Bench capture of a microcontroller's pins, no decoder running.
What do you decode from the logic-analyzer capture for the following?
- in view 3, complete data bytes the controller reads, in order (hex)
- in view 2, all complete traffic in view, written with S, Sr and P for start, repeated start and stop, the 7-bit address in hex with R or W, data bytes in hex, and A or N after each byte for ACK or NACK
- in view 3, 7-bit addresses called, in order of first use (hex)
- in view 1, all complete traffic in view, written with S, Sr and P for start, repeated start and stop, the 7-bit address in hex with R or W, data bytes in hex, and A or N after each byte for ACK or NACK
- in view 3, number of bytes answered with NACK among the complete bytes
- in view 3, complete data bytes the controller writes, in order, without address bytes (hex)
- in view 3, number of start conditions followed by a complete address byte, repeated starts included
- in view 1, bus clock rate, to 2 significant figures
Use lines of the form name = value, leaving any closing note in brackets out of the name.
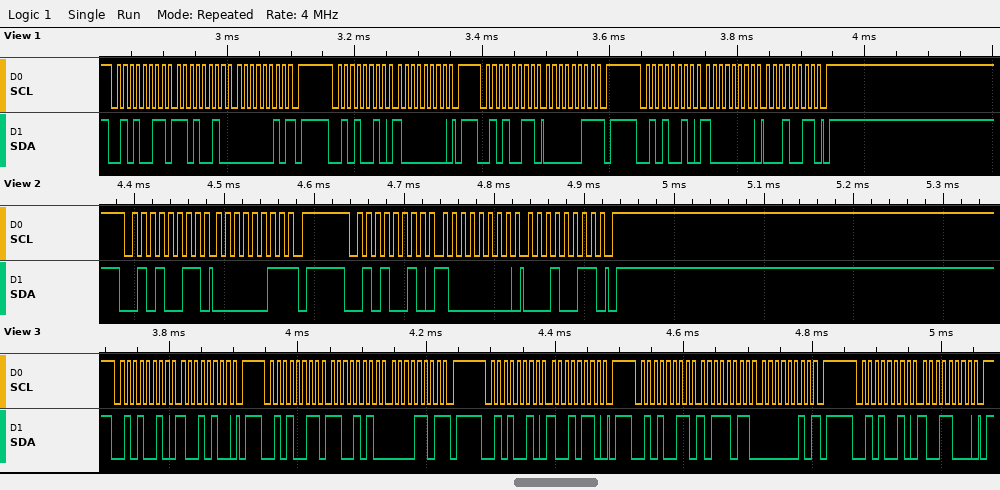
in view 3, complete data bytes the controller reads, in order = CA 0D BB 02
in view 2, all complete traffic in view, written with S, Sr and P for start, repeated start and stop, the 7-bit address in hex with R or W, data bytes in hex, and A or N after each byte for ACK or NACK = S 29R A 03 N P S 29W A 80 A 13 A P
in view 3, 7-bit addresses called, in order of first use = 0x29
in view 1, all complete traffic in view, written with S, Sr and P for start, repeated start and stop, the 7-bit address in hex with R or W, data bytes in hex, and A or N after each byte for ACK or NACK = S 29R A D2 A 02 N P S 29W A 80 A P S 29R A 03 N P S 29W A 80 A 13 A P
in view 3, number of bytes answered with NACK among the complete bytes = 2
in view 3, complete data bytes the controller writes, in order, without address bytes = 94 96 98
in view 3, number of start conditions followed by a complete address byte, repeated starts included = 5
in view 1, bus clock rate, to 2 significant figures = 100 kHz
